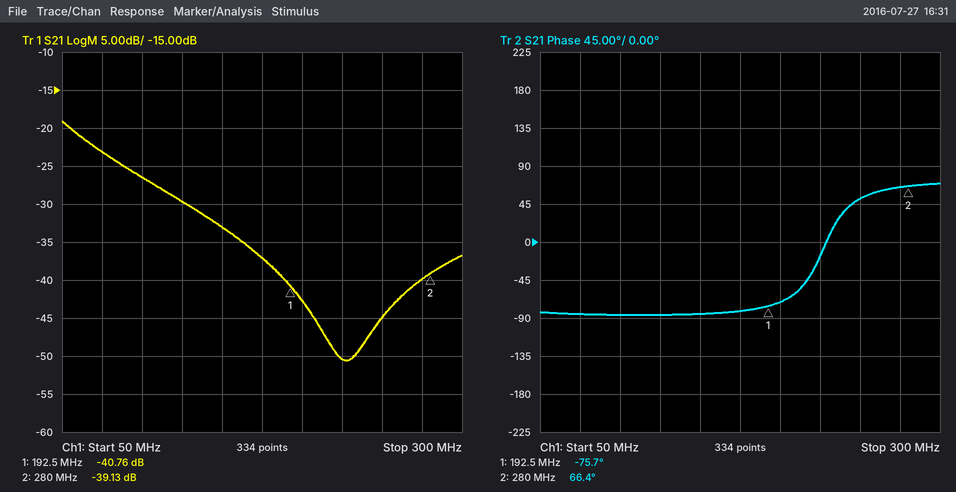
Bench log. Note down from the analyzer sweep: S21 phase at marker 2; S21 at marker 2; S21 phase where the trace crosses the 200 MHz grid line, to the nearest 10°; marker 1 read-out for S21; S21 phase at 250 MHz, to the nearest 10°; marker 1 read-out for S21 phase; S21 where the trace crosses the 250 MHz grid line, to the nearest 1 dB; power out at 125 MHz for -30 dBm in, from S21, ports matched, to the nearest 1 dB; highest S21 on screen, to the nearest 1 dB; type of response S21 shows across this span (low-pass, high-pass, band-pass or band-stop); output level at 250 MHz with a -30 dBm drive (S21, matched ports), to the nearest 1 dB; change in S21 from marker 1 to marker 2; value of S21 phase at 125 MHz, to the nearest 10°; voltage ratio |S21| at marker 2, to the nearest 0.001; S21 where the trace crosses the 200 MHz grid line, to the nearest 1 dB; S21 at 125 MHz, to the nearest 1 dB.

66.4°
-39.13 dB
-70°
-40.76 dB
50°
-75.7°
-45 dB
-60 dBm
-19 dB
low-pass
-75 dBm
1.63 dB
-90°
0.011
-43 dB
-30 dB
